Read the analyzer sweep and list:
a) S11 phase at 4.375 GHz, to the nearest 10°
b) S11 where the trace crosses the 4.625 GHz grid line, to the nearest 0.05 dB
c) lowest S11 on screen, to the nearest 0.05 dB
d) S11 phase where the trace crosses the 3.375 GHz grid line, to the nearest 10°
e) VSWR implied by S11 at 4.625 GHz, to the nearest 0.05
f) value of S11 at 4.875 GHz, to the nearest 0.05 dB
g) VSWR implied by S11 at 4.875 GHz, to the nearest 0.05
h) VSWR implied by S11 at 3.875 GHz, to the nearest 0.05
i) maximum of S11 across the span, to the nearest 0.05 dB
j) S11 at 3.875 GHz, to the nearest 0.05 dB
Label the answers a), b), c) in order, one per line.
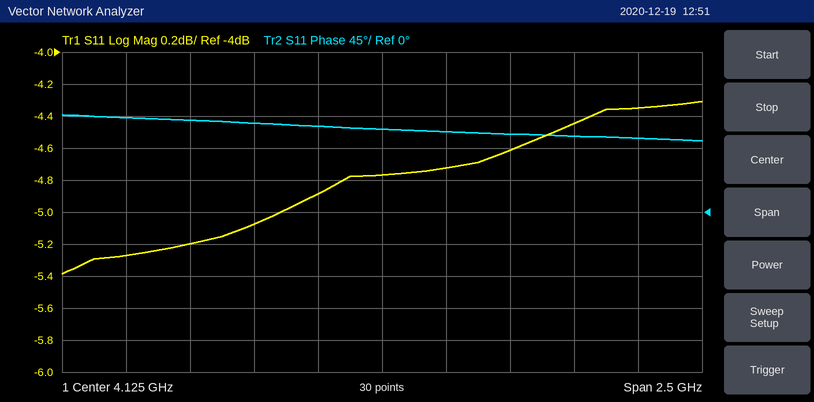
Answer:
a) 110°
b) -4.60 dB
c) -5.40 dB
d) 130°
e) 3.85
f) -4.45 dB
g) 4.00
h) 3.65
i) -4.30 dB
j) -4.90 dB
